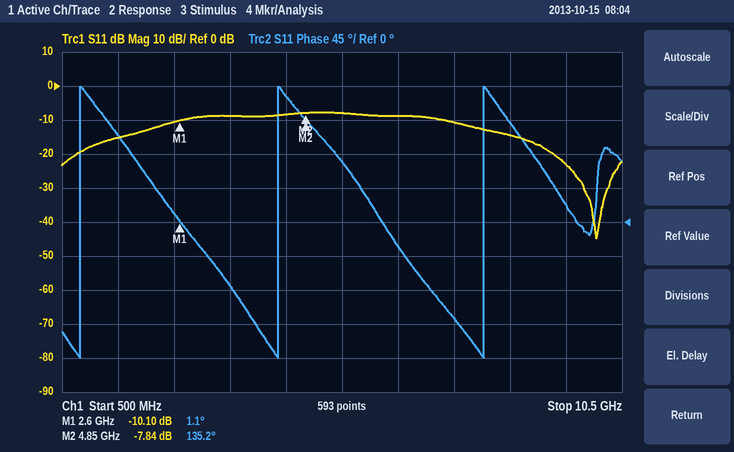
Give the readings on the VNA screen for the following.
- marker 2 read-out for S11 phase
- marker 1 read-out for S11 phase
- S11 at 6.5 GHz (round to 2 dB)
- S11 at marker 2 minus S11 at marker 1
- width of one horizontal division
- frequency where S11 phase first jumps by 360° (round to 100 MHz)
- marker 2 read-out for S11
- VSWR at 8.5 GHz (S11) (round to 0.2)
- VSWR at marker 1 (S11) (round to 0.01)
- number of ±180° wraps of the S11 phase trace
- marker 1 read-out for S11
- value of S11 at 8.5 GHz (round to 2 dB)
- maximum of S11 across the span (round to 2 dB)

135.2°
1.1°
-8 dB
2.26 dB
1 GHz
800 MHz
-7.84 dB
1.4
1.91
3
-10.10 dB
-14 dB
-8 dB
